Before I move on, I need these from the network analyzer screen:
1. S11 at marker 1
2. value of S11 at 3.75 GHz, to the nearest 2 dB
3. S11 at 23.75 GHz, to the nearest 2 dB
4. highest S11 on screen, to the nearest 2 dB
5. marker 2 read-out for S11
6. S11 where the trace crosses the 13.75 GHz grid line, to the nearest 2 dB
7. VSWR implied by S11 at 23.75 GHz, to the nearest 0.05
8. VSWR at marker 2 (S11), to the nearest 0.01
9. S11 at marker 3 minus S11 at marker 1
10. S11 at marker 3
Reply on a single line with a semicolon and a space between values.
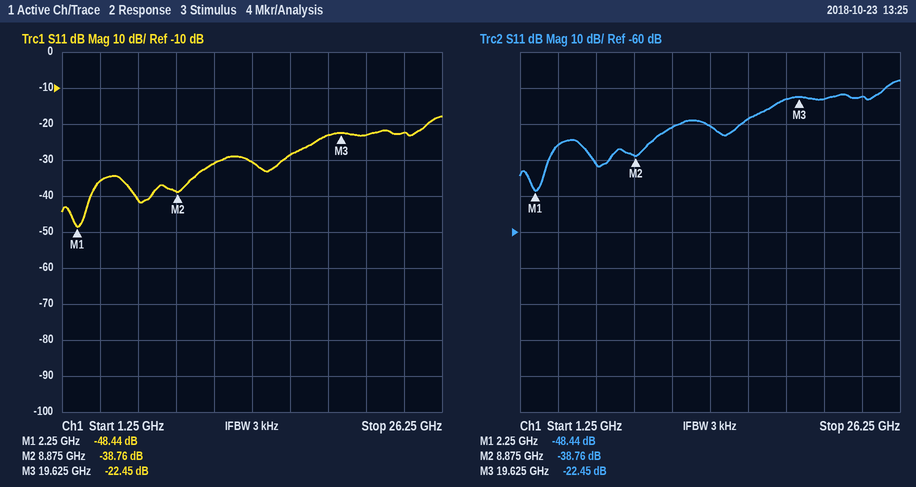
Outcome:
-48.44 dB; -36 dB; -22 dB; -18 dB; -38.76 dB; -30 dB; 1.15; 1.02; 25.99 dB; -22.45 dB
